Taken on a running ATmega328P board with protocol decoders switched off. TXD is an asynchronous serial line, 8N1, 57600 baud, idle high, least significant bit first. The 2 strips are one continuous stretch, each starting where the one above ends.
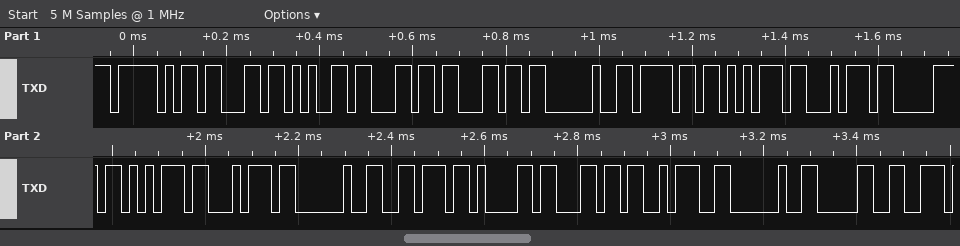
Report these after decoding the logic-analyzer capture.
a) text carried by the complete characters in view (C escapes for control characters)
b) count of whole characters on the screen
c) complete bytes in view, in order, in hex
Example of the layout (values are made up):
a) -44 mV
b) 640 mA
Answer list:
a) "_cell output val: 0"
b) 19
c) 5F 63 65 6C 6C 20 6F 75 74 70 75 74 20 76 61 6C 3A 20 30
